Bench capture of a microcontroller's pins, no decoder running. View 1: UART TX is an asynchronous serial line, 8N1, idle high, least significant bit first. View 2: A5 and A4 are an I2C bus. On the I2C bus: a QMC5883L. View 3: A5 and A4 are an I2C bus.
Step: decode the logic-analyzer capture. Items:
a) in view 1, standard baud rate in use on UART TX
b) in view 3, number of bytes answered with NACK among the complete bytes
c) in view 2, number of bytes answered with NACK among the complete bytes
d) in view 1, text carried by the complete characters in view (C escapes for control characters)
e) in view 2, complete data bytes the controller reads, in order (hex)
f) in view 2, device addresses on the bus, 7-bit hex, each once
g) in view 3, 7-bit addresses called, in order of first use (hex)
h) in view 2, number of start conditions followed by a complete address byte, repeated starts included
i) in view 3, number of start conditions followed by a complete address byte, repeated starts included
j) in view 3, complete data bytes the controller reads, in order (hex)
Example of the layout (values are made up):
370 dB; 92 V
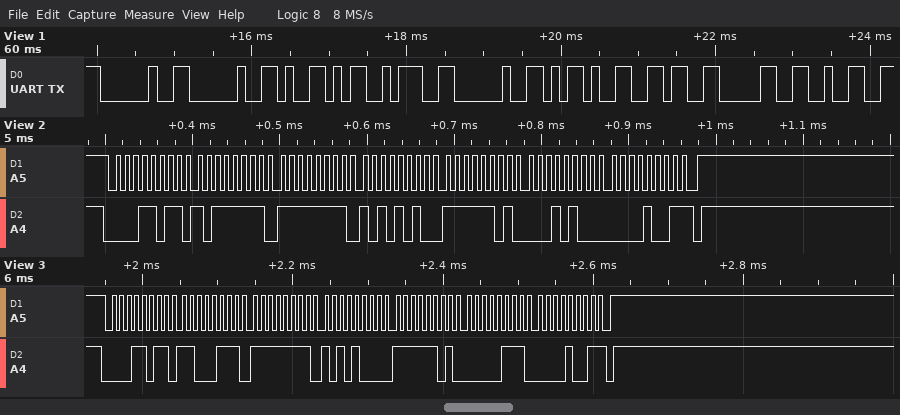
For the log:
9600 baud; 1; 1; "  Y: -602"; BF FF AA FD 14 09; 0x0D; 0x0D; 1; 1; C7 FF A8 FD 07 09
